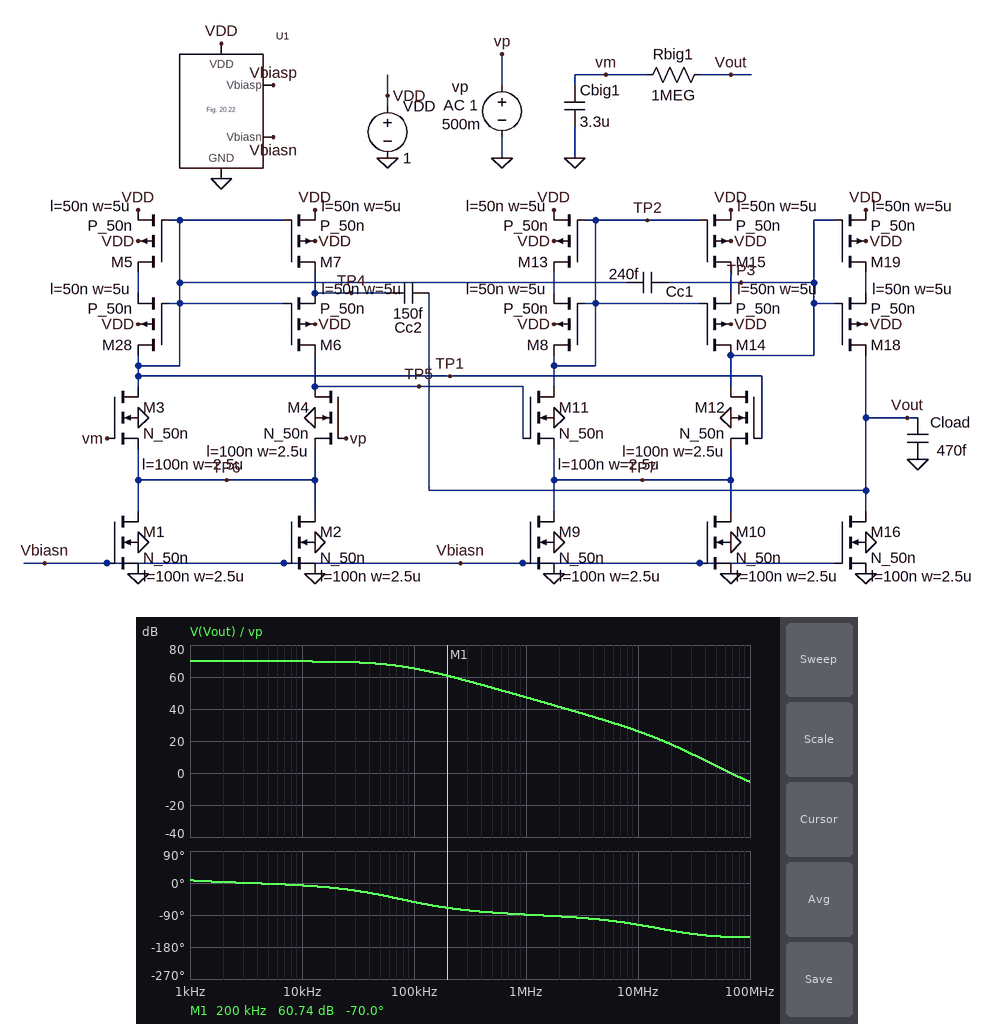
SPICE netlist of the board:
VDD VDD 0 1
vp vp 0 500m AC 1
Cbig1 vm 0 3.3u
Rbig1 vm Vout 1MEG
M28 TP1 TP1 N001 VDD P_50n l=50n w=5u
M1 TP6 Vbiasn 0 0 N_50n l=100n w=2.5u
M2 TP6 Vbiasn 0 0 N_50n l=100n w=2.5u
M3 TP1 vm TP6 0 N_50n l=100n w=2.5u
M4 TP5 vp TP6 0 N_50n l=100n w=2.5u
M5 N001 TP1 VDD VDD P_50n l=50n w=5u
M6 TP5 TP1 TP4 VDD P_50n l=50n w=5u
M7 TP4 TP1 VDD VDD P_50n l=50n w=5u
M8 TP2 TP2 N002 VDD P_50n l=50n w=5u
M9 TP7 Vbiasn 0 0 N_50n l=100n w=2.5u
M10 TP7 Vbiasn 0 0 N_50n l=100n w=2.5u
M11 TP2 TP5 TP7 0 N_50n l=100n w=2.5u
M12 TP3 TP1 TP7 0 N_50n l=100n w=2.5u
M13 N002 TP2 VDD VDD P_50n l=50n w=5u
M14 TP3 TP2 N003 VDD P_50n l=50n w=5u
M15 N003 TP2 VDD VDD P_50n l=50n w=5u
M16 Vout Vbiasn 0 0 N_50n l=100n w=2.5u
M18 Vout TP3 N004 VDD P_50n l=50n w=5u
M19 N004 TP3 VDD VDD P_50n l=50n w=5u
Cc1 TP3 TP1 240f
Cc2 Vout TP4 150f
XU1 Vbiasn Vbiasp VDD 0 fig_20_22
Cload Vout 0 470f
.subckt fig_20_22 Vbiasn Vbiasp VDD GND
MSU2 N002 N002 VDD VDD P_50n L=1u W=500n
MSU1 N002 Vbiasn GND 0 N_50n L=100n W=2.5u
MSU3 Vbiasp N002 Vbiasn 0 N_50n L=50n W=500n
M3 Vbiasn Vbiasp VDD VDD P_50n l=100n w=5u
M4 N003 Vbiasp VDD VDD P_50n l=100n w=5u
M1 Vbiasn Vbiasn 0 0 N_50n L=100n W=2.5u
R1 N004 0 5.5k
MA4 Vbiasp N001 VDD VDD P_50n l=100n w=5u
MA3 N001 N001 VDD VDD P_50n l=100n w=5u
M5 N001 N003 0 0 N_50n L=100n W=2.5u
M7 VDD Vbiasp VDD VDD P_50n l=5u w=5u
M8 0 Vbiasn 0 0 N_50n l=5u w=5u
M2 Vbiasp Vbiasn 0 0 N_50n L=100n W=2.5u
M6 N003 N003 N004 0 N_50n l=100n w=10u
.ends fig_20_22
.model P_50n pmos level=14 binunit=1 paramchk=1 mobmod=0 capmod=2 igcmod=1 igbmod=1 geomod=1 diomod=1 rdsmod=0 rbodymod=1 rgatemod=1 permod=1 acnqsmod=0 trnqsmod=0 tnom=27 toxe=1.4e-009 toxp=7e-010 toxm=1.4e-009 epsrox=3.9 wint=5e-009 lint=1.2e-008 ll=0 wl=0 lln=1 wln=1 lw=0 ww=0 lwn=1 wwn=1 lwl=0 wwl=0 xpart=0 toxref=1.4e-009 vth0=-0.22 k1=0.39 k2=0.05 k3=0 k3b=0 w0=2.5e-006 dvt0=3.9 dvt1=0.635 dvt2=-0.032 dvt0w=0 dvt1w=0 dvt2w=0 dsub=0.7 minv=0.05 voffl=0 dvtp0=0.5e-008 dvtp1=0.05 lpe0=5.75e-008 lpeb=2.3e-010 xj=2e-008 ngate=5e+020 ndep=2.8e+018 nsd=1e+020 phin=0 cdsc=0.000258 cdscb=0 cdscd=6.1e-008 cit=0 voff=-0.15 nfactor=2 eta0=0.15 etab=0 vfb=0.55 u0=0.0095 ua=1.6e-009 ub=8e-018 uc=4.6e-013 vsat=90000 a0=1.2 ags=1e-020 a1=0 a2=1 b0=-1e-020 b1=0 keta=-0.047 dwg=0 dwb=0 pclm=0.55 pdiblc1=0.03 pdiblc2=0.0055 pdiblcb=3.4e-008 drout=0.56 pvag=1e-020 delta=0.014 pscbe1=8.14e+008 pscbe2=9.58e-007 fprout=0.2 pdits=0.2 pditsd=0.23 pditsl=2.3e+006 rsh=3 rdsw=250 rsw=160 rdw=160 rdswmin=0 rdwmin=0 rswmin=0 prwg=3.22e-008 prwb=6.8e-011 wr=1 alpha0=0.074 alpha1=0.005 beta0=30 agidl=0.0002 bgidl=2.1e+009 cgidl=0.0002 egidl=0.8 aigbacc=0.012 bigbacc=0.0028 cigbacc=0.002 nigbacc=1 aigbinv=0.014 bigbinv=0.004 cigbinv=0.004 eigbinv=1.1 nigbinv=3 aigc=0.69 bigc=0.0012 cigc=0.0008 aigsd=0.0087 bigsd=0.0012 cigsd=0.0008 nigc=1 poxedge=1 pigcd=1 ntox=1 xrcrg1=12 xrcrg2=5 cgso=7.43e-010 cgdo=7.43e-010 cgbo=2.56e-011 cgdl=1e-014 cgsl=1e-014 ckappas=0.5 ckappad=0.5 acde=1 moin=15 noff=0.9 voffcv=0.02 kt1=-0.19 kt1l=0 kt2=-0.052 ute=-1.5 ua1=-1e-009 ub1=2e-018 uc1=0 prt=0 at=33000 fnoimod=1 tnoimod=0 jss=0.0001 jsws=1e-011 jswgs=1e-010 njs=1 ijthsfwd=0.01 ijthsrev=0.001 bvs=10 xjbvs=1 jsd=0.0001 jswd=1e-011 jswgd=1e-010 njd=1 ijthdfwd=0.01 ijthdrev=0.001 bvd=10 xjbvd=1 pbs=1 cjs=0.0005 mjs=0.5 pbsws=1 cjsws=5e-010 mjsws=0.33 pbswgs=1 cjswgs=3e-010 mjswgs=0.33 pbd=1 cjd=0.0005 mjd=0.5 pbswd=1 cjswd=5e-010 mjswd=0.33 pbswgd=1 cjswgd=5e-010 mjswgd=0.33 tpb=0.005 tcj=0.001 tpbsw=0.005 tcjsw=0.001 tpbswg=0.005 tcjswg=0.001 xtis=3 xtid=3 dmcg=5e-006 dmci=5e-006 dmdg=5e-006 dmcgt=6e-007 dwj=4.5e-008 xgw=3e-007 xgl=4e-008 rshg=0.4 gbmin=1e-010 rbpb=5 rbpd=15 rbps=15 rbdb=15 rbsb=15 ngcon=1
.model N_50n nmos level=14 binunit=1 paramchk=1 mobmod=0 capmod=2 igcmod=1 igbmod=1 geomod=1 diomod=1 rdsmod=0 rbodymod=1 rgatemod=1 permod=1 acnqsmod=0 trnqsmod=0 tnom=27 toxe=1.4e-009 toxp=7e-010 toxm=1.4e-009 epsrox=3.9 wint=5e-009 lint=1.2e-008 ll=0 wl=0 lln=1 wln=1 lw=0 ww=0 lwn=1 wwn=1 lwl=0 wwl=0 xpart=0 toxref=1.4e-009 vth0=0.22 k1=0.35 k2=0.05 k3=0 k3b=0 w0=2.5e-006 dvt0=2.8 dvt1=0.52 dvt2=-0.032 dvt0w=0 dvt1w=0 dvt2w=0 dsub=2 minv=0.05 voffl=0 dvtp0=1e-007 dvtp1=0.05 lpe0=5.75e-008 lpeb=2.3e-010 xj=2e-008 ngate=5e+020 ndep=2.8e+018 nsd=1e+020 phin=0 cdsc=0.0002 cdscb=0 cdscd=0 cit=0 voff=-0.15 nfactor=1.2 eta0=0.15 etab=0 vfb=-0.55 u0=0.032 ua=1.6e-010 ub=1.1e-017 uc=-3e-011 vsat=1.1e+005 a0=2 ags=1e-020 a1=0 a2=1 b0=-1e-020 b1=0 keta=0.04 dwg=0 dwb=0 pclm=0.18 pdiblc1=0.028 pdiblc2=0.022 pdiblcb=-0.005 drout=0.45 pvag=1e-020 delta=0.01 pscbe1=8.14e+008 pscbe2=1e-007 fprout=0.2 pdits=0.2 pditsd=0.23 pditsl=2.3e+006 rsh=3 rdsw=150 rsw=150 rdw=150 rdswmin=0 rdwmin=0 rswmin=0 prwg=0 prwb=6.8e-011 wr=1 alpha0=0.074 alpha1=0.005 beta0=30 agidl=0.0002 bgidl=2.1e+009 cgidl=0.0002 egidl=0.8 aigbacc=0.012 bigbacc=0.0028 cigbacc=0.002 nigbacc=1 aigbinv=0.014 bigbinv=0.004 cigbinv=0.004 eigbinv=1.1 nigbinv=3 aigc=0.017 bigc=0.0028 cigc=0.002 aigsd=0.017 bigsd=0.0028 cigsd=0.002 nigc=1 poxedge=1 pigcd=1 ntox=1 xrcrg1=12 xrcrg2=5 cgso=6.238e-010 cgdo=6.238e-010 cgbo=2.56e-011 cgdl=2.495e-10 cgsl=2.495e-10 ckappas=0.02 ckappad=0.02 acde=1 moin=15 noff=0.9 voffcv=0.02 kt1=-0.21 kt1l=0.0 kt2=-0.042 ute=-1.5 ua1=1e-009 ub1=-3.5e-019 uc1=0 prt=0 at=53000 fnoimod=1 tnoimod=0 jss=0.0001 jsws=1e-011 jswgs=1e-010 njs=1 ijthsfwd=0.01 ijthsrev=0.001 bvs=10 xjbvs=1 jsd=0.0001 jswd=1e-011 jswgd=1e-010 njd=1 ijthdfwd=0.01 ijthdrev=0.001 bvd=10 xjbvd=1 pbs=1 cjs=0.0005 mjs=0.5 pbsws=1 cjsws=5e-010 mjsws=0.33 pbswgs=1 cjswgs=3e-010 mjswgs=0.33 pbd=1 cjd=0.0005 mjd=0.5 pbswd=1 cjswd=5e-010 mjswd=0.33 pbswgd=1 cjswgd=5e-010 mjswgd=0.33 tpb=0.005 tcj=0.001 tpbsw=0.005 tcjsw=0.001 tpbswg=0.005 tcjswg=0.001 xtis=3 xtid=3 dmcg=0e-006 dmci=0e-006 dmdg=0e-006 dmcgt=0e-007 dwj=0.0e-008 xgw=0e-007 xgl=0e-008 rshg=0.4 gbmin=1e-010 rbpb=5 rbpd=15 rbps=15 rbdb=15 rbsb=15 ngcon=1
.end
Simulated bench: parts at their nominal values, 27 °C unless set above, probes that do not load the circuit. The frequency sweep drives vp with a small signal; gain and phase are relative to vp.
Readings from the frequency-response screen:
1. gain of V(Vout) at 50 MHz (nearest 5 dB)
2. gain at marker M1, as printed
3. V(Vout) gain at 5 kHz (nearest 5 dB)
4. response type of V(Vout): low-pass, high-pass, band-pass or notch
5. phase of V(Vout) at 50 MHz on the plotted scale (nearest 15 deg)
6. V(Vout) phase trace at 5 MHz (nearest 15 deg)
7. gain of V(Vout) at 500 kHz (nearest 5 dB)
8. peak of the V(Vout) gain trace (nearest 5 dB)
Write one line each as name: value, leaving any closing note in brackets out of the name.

gain of V(Vout) at 50 MHz: 5 dB
gain at marker M1, as printed: 60.74 dB
V(Vout) gain at 5 kHz: 70 dB
response type of V(Vout): low-pass, high-pass, band-pass or notch: low-pass
phase of V(Vout) at 50 MHz on the plotted scale: -150 deg
V(Vout) phase trace at 5 MHz: -105 deg
gain of V(Vout) at 500 kHz: 55 dB
peak of the V(Vout) gain trace: 70 dB
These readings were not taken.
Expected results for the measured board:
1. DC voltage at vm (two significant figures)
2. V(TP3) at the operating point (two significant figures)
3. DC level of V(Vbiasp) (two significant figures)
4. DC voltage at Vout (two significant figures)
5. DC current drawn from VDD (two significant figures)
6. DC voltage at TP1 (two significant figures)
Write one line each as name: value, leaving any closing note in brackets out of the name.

DC voltage at vm: 500 mV
V(TP3) at the operating point: 670 mV
DC level of V(Vbiasp): 650 mV
DC voltage at Vout: 500 mV
DC current drawn from VDD: 96 µA
DC voltage at TP1: 680 mV
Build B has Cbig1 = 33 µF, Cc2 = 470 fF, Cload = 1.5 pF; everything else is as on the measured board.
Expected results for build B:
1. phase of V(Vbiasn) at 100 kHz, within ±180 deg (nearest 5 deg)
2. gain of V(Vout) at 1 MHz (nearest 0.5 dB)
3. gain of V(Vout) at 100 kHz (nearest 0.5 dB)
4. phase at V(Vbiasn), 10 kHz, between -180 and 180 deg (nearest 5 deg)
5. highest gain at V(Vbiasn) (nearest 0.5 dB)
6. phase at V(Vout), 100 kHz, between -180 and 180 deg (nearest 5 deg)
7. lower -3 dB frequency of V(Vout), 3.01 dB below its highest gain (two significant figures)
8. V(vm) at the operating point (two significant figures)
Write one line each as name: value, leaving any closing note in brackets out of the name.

phase of V(Vbiasn) at 100 kHz, within ±180 deg: 10 deg
gain of V(Vout) at 1 MHz: 38.5 dB
gain of V(Vout) at 100 kHz: 58.0 dB
phase at V(Vbiasn), 10 kHz, between -180 and 180 deg: 30 deg
highest gain at V(Vbiasn): -39.0 dB
phase at V(Vout), 100 kHz, between -180 and 180 deg: -75 deg
lower -3 dB frequency of V(Vout), 3.01 dB below its highest gain: 15 Hz
V(vm) at the operating point: 500 mV
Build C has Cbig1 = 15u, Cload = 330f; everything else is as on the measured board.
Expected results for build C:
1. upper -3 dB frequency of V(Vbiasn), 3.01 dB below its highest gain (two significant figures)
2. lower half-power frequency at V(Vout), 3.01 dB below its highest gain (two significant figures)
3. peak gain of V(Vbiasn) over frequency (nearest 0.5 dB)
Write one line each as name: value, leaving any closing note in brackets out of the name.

upper -3 dB frequency of V(Vbiasn), 3.01 dB below its highest gain: 12 MHz
lower half-power frequency at V(Vout), 3.01 dB below its highest gain: 33 Hz
peak gain of V(Vbiasn) over frequency: -30.0 dB
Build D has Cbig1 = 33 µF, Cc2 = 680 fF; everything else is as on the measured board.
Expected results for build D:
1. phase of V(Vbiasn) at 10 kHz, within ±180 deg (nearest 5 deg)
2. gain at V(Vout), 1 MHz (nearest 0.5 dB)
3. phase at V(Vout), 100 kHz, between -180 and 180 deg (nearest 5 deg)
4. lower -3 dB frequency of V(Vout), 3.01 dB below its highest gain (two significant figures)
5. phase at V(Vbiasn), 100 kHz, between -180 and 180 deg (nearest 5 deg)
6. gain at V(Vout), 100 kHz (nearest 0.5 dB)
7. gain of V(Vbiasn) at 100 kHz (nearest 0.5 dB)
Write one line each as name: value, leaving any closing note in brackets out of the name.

phase of V(Vbiasn) at 10 kHz, within ±180 deg: 25 deg
gain at V(Vout), 1 MHz: 35.5 dB
phase at V(Vout), 100 kHz, between -180 and 180 deg: -80 deg
lower -3 dB frequency of V(Vout), 3.01 dB below its highest gain: 15 Hz
phase at V(Vbiasn), 100 kHz, between -180 and 180 deg: 5 deg
gain at V(Vout), 100 kHz: 55.5 dB
gain of V(Vbiasn) at 100 kHz: -42.0 dB
